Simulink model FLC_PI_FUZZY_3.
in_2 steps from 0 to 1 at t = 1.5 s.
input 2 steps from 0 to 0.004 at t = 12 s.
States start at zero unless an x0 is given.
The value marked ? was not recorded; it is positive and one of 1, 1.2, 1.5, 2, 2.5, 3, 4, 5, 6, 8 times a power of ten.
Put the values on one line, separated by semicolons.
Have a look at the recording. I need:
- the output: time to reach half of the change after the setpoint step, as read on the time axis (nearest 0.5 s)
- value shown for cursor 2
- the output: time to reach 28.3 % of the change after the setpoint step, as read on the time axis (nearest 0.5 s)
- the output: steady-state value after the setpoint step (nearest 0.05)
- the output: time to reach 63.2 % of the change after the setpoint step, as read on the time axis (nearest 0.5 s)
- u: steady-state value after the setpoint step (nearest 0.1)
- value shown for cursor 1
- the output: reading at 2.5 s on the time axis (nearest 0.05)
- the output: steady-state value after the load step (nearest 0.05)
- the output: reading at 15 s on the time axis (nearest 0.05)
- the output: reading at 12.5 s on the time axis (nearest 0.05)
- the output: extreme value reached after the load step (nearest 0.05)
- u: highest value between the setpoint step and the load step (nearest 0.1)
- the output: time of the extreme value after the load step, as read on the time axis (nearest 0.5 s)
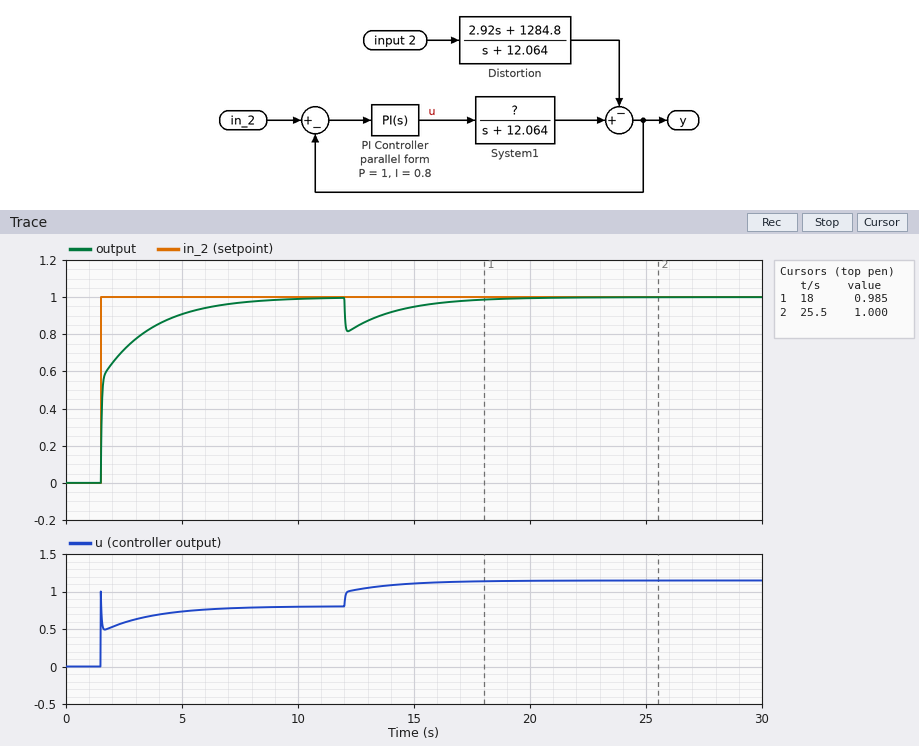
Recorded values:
1.5 s; 1.000; 1.5 s; 1.00; 2.0 s; 0.8; 0.985; 0.70; 1.00; 0.95; 0.85; 0.80; 1.0; 12.0 s
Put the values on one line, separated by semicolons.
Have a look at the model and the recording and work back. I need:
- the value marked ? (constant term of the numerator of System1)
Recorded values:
15
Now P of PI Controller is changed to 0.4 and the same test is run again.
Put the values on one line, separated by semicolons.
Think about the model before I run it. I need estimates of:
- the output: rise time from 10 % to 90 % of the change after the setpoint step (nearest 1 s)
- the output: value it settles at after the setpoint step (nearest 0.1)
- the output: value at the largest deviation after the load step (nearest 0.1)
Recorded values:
3 s; 1.0; 0.7
